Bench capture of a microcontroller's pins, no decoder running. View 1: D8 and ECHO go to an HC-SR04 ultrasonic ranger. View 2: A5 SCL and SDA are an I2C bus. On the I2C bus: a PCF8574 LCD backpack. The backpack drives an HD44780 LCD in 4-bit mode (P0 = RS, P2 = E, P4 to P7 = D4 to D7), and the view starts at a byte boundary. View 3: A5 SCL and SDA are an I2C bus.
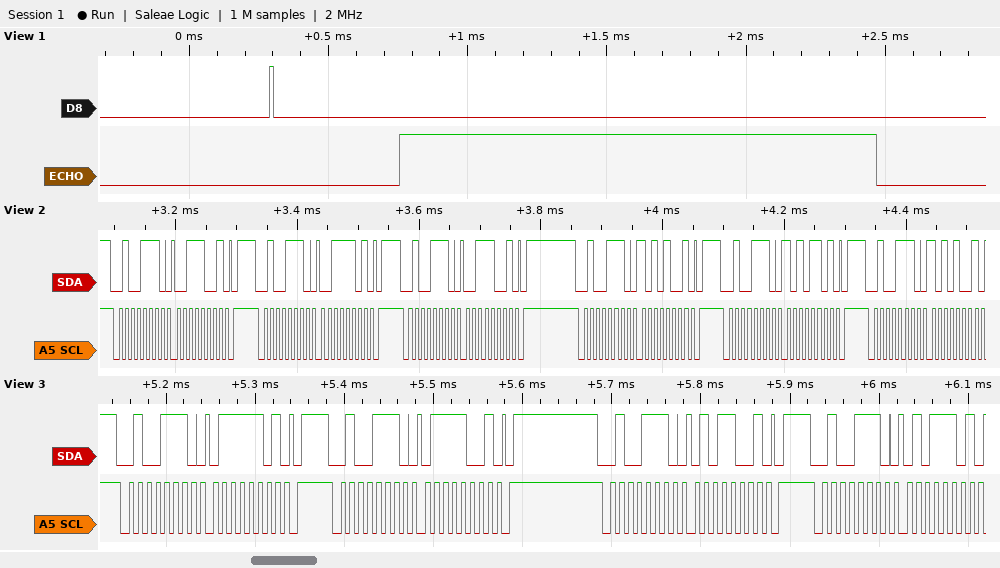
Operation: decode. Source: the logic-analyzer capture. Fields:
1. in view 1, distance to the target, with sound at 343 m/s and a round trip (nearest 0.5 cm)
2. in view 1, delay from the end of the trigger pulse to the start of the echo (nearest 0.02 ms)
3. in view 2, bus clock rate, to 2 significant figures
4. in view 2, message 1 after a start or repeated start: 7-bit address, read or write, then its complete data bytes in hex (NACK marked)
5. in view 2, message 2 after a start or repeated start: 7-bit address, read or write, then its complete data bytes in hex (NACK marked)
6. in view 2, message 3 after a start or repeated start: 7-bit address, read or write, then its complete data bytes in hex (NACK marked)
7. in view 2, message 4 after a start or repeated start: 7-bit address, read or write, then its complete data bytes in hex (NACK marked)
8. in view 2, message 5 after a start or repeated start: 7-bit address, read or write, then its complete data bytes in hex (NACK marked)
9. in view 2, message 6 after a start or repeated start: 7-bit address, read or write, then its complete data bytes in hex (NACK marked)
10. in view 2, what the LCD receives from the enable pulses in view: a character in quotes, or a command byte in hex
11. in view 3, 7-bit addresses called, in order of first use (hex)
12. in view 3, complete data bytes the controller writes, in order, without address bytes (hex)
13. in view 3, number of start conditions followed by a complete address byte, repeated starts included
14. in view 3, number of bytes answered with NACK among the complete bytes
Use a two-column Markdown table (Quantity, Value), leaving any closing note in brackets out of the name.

| Quantity | Value |
|---|---|
| in view 1, distance to the target, with sound at 343 m/s and a round trip | 29.5 cm |
| in view 1, delay from the end of the trigger pulse to the start of the echo | 0.46 ms |
| in view 2, bus clock rate, to 2 significant figures | 100 kHz |
| in view 2, message 1 after a start or repeated start: 7-bit address, read or write, then its complete data bytes in hex | 0x27 write: 39 |
| in view 2, message 2 after a start or repeated start: 7-bit address, read or write, then its complete data bytes in hex | 0x27 write: 3D |
| in view 2, message 3 after a start or repeated start: 7-bit address, read or write, then its complete data bytes in hex | 0x27 write: 39 |
| in view 2, message 4 after a start or repeated start: 7-bit address, read or write, then its complete data bytes in hex | 0x27 write: A9 |
| in view 2, message 5 after a start or repeated start: 7-bit address, read or write, then its complete data bytes in hex | 0x27 write: AD |
| in view 2, message 6 after a start or repeated start: 7-bit address, read or write, then its complete data bytes in hex | 0x27 write: A9 |
| in view 2, what the LCD receives from the enable pulses in view: a character in quotes, or a command byte in hex | ':' |
| in view 3, 7-bit addresses called, in order of first use | 0x27 |
| in view 3, complete data bytes the controller writes, in order, without address bytes | 7D 79 59 5D |
| in view 3, number of start conditions followed by a complete address byte, repeated starts included | 4 |
| in view 3, number of bytes answered with NACK among the complete bytes | 0 |
